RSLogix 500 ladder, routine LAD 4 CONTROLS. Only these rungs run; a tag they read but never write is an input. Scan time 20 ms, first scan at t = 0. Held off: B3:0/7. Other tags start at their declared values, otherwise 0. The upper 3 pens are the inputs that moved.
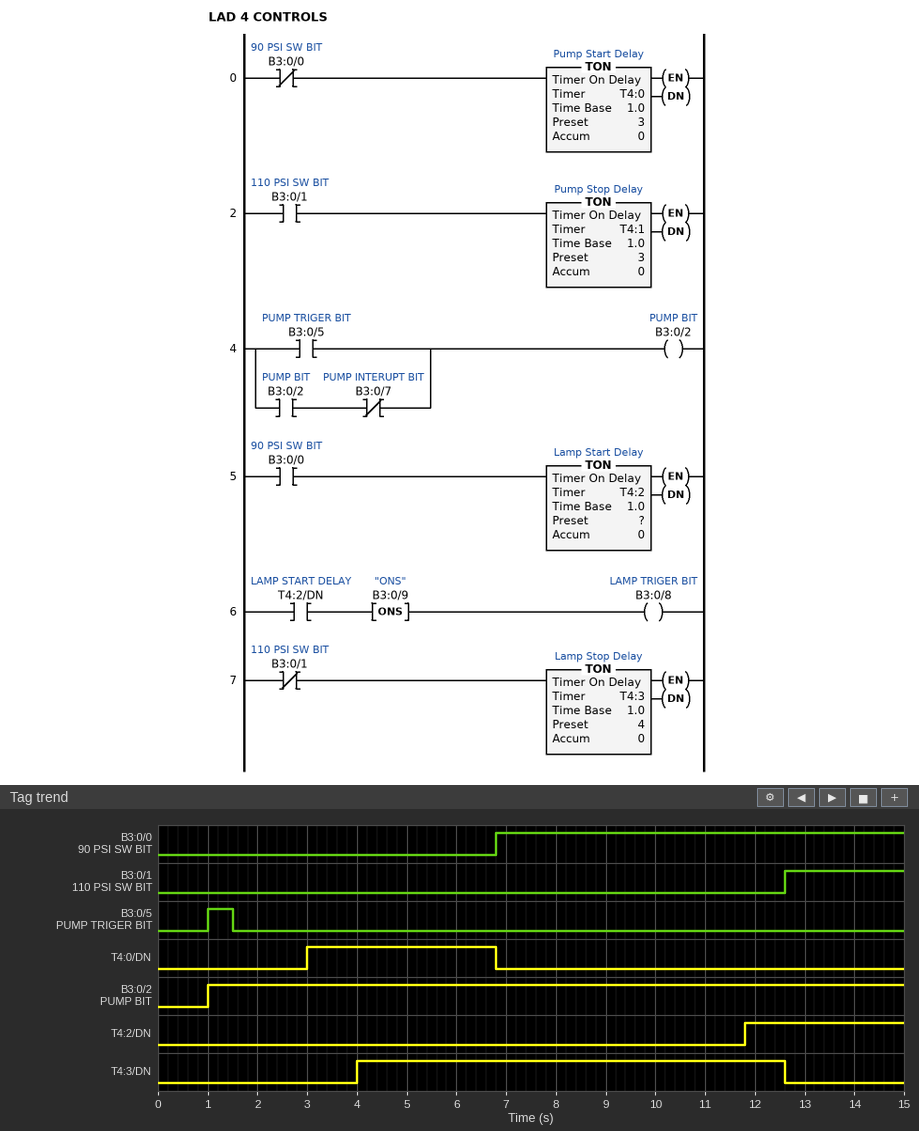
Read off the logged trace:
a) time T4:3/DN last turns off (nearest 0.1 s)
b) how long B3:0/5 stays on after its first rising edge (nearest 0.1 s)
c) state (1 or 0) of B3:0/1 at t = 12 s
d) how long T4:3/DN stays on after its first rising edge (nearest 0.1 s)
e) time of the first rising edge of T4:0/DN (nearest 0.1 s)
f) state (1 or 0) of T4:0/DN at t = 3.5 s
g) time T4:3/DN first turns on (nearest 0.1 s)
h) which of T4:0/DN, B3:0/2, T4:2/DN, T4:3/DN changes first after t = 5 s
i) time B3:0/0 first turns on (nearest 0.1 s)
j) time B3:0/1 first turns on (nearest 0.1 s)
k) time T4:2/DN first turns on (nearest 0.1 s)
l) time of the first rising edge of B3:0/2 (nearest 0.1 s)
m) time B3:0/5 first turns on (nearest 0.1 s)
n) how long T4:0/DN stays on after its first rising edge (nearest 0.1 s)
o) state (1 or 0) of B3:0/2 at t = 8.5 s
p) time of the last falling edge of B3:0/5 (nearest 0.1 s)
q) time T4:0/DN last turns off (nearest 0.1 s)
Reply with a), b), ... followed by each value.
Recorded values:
a) 12.6 s
b) 0.5 s
c) 0
d) 8.6 s
e) 3.0 s
f) 1
g) 4.0 s
h) T4:0/DN
i) 6.8 s
j) 12.6 s
k) 11.8 s
l) 1.0 s
m) 1.0 s
n) 3.8 s
o) 1
p) 1.5 s
q) 6.8 s
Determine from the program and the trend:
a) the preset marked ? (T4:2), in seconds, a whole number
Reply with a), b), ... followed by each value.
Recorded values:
a) 5 s
